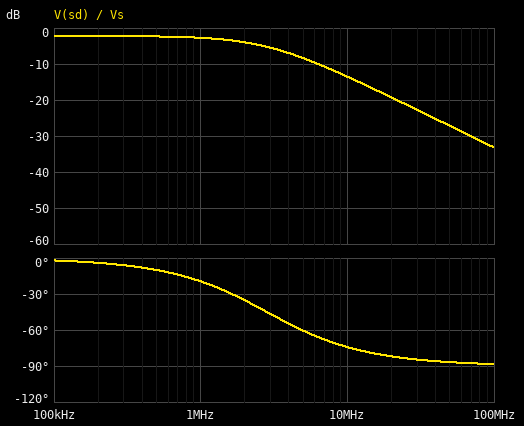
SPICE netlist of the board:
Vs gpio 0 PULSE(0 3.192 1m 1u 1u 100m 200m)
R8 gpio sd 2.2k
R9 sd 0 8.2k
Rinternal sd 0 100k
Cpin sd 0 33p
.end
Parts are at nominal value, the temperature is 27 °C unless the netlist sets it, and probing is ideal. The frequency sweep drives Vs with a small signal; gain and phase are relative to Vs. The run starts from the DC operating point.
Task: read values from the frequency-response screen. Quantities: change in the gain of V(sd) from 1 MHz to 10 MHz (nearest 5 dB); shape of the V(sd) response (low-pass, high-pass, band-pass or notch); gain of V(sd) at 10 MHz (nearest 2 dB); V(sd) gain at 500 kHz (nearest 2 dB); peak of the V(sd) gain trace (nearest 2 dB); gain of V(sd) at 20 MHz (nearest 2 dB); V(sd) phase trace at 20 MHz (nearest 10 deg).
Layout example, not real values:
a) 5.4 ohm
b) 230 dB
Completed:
a) -10 dB
b) low-pass
c) -14 dB
d) -2 dB
e) -2 dB
f) -20 dB
g) -80 deg
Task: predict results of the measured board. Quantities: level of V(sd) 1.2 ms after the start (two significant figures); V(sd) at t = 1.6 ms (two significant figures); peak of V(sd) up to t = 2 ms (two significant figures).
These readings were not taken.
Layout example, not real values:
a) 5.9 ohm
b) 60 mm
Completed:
a) 2.5 V
b) 2.5 V
c) 2.5 V
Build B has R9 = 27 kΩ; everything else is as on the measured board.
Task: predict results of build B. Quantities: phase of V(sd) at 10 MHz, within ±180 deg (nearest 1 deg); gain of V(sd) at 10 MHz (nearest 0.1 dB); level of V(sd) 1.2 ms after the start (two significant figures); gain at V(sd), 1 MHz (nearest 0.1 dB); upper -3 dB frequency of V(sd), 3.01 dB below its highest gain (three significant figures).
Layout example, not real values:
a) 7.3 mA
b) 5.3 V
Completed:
a) -76 deg
b) -13.4 dB
c) 2.9 V
d) -1.5 dB
e) 2.42 MHz
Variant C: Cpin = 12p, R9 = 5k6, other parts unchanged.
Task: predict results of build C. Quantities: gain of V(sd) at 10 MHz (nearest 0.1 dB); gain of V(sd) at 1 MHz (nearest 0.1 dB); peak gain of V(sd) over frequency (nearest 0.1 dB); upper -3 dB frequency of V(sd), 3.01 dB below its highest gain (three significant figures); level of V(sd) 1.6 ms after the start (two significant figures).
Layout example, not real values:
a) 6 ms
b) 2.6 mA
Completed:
a) -6.8 dB
b) -3.1 dB
c) -3.0 dB
d) 8.53 MHz
e) 2.3 V
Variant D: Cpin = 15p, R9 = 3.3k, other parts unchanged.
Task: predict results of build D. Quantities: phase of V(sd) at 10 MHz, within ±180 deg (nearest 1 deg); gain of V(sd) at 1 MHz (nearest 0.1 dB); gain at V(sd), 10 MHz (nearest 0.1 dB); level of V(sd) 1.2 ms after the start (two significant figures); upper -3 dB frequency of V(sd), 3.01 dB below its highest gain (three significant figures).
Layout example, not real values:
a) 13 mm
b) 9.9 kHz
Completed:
a) -51 deg
b) -4.6 dB
c) -8.5 dB
d) 1.9 V
e) 8.14 MHz
